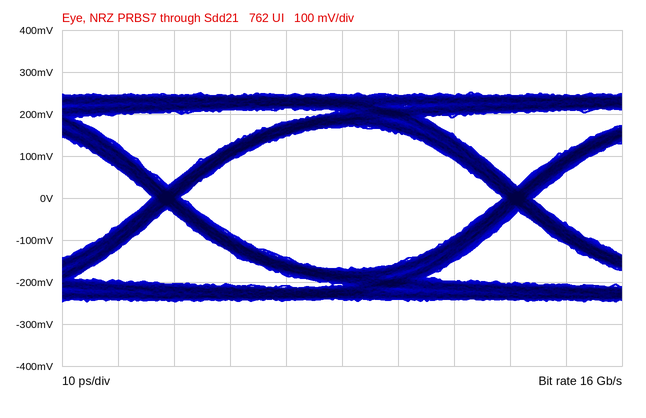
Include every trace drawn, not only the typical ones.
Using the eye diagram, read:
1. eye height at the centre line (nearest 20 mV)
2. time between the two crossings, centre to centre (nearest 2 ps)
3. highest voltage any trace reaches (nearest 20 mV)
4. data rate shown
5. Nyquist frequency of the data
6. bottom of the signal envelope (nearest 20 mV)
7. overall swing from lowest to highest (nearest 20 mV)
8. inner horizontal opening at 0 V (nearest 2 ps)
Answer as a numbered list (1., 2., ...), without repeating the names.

1. 340 mV
2. 62 ps
3. 260 mV
4. 16 Gb/s
5. 8 GHz
6. -240 mV
7. 500 mV
8. 58 ps
